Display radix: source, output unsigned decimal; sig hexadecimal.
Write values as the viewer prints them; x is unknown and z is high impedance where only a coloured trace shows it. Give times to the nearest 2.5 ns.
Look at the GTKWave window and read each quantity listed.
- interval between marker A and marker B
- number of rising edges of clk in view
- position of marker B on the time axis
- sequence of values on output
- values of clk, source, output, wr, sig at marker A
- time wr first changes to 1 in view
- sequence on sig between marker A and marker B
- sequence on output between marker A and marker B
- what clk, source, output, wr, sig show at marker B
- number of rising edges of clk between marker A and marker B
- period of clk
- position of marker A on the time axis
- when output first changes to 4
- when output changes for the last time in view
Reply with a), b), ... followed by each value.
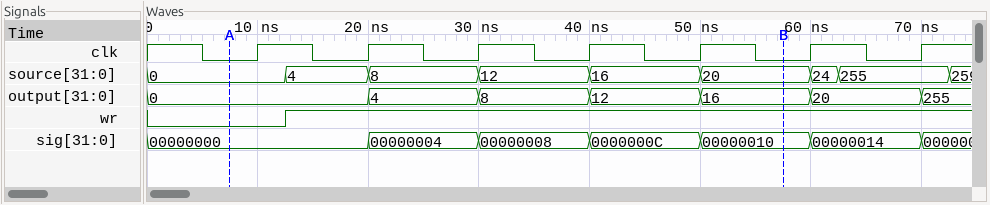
a) 50 ns
b) 7
c) 57.5 ns
d) 0, 4, 8, 12, 16, 20, 255
e) clk=0, source=0, output=0, wr=0, sig=00000000
f) 12.5 ns
g) 00000000, 00000004, 00000008, 0000000C, 00000010
h) 0, 4, 8, 12, 16
i) clk=0, source=20, output=16, wr=1, sig=00000010
j) 5
k) 10 ns
l) 7.5 ns
m) 20 ns
n) 70 ns
